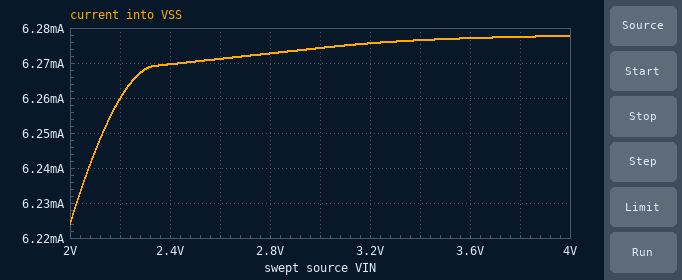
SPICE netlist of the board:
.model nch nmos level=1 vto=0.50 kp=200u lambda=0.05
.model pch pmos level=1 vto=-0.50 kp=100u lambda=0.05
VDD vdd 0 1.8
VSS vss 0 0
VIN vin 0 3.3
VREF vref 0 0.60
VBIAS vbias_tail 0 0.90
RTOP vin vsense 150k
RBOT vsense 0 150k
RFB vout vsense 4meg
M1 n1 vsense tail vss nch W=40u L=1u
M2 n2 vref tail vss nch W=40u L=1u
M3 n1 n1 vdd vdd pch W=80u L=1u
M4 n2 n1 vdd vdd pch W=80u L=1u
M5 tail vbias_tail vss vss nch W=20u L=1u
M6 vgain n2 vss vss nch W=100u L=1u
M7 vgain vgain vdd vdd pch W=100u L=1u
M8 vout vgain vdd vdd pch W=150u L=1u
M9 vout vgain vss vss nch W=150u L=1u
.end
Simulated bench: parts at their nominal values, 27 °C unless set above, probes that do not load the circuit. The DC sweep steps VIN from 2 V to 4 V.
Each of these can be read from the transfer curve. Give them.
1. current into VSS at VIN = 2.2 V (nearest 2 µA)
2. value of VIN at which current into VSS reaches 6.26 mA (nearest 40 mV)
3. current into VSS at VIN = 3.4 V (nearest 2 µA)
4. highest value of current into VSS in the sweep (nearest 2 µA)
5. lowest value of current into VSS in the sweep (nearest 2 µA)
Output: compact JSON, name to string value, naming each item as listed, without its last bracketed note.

{"current into VSS at VIN = 2.2 V": "6.260 mA", "value of VIN at which current into VSS reaches 6.26 mA": "2.20 V", "current into VSS at VIN = 3.4 V": "6.276 mA", "highest value of current into VSS in the sweep": "6.278 mA", "lowest value of current into VSS in the sweep": "6.224 mA"}
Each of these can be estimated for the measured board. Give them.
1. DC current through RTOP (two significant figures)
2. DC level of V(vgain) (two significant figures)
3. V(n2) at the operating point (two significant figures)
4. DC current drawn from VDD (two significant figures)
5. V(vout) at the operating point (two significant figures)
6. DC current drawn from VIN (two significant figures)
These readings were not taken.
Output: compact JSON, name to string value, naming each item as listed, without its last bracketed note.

{"DC current through RTOP": "11 µA", "DC level of V(vgain)": "250 mV", "V(n2) at the operating point": "1.8 V", "DC current drawn from VDD": "6.3 mA", "V(vout) at the operating point": "1.8 V", "DC current drawn from VIN": "11 µA"}
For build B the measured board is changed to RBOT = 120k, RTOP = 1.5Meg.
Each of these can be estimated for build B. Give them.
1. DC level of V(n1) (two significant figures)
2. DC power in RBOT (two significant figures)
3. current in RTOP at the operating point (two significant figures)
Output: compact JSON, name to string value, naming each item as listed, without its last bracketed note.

{"DC level of V(n1)": "1.3 V", "DC power in RBOT": "470 nW", "current in RTOP at the operating point": "2.0 µA"}
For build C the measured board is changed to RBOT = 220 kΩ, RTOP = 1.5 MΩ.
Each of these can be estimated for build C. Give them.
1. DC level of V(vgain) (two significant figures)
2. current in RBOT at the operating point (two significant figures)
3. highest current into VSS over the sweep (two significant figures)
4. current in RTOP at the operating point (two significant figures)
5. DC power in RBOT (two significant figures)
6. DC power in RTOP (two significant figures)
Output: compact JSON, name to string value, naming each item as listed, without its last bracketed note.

{"DC level of V(vgain)": "1.3 V", "current in RBOT at the operating point": "1.8 µA", "highest current into VSS over the sweep": "120 nA", "current in RTOP at the operating point": "1.9 µA", "DC power in RBOT": "740 nW", "DC power in RTOP": "5.6 µW"}
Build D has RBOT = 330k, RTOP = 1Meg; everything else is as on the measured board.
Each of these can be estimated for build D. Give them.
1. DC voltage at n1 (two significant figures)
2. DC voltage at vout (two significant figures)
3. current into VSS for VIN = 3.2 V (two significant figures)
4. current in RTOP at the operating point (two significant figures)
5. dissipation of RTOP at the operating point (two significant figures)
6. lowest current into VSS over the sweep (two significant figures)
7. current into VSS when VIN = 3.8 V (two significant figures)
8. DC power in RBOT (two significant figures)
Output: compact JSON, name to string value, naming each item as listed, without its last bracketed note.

{"DC voltage at n1": "1.1 V", "DC voltage at vout": "1.8 V", "current into VSS for VIN = 3.2 V": "6.1 mA", "current in RTOP at the operating point": "2.4 µA", "dissipation of RTOP at the operating point": "5.9 µW", "lowest current into VSS over the sweep": "120 nA", "current into VSS when VIN = 3.8 V": "6.2 mA", "DC power in RBOT": "2.3 µW"}
